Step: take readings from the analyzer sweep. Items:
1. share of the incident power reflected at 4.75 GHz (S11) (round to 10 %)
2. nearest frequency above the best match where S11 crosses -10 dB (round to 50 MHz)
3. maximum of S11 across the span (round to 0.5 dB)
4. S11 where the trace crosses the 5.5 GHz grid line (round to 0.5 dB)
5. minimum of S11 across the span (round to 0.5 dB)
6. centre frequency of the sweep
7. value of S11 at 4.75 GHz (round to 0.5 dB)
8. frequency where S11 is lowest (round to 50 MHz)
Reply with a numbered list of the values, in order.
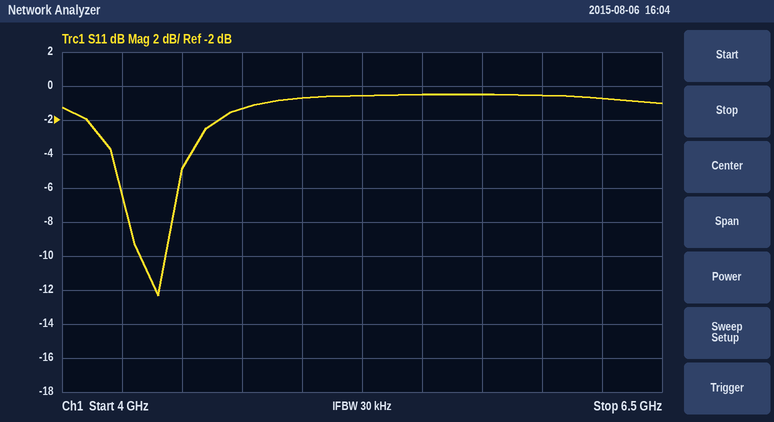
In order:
1. 70 %
2. 4.45 GHz
3. -0.5 dB
4. -0.5 dB
5. -12.5 dB
6. 5.25 GHz
7. -1.5 dB
8. 4.40 GHz
